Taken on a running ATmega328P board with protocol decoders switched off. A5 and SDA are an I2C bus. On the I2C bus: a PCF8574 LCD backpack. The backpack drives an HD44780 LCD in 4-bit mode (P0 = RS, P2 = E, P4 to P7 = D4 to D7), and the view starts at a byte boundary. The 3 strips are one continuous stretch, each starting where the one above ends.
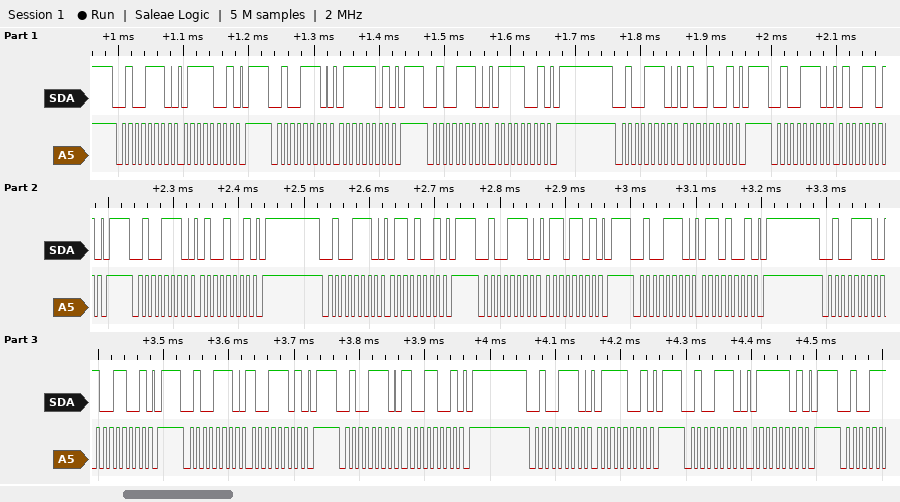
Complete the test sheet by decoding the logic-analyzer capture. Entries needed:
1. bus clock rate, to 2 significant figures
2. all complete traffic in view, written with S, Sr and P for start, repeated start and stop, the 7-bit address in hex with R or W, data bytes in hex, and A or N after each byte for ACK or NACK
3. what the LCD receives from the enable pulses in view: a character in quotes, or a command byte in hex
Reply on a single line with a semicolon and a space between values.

100 kHz; S 27W A 79 A P S 27W A 7D A P S 27W A 79 A P S 27W A 49 A P S 27W A 4D A P S 27W A 49 A P S 27W A 69 A P S 27W A 6D A P S 27W A 69 A P S 27W A 99 A P S 27W A 9D A P S 27W A 99 A P S 27W A 79 A P S 27W A 7D A P; 't' 'i'
